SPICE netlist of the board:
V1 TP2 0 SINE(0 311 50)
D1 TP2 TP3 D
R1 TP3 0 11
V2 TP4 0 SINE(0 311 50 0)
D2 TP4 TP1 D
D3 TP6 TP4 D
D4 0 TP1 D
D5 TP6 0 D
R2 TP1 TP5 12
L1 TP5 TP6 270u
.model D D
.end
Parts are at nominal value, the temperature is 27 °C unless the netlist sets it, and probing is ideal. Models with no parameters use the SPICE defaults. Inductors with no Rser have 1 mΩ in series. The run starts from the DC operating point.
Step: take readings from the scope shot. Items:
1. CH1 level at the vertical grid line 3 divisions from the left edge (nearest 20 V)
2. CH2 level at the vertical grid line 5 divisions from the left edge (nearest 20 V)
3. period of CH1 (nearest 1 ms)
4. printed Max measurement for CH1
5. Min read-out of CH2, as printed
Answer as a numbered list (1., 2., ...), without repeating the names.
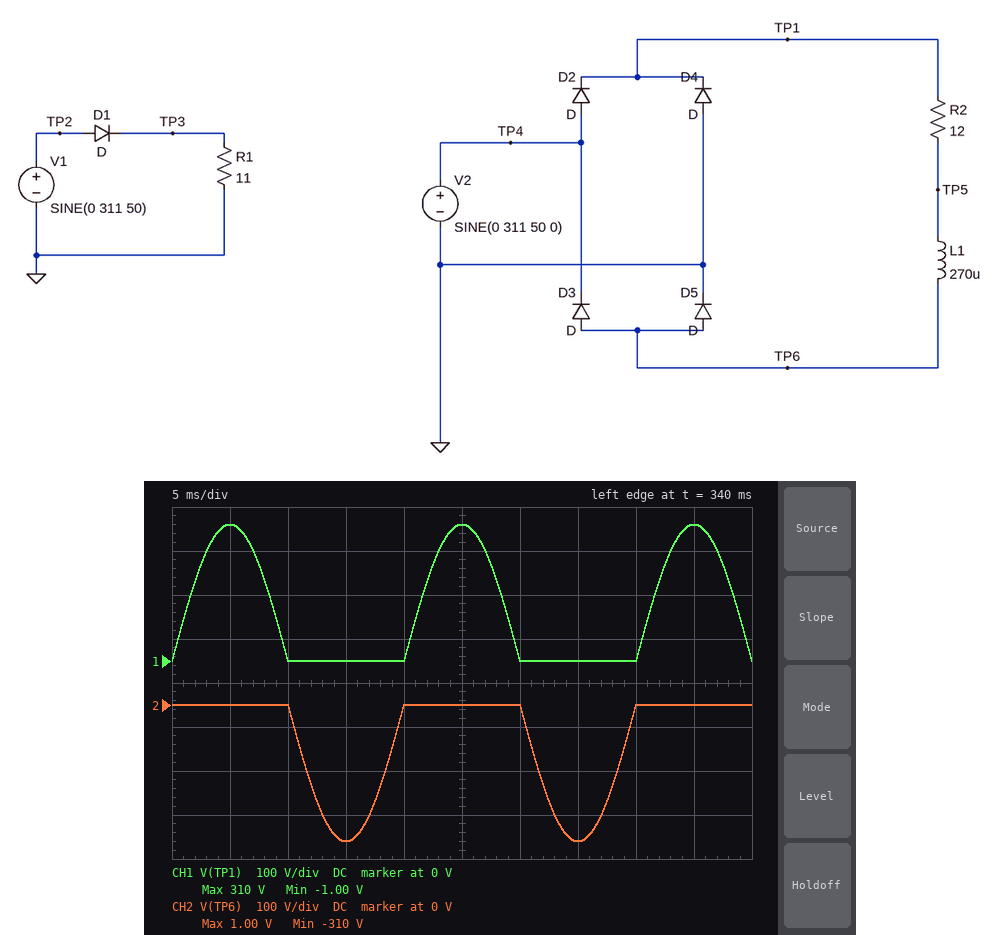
1. 0 V
2. 0 V
3. 20 ms
4. 310 V
5. -310 V
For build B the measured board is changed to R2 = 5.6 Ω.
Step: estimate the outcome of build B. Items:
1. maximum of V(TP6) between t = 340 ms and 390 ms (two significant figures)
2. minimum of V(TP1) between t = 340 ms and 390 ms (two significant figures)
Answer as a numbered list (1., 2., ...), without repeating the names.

1. 940 mV
2. -940 mV
